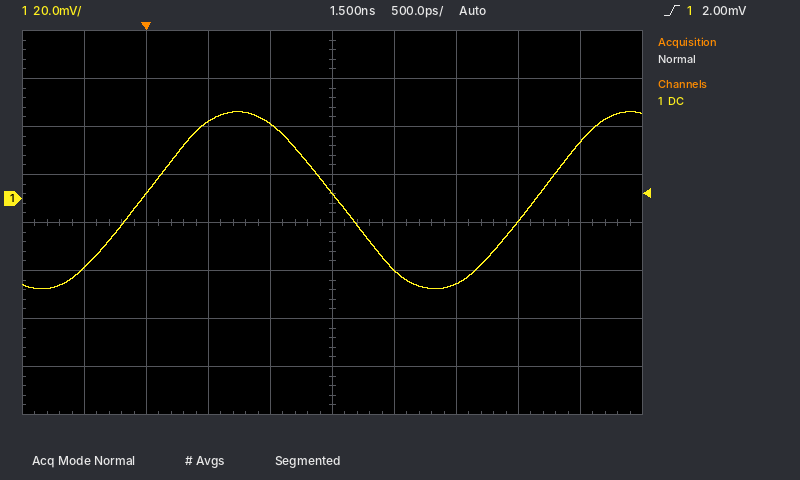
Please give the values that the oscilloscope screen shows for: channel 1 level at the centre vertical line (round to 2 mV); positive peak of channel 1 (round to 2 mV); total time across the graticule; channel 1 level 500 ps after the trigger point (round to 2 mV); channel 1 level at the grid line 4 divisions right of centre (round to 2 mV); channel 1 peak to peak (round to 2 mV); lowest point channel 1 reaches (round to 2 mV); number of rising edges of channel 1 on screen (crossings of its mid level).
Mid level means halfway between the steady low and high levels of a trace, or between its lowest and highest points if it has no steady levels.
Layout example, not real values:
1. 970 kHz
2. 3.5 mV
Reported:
1. 2 mV
2. 36 mV
3. 5 ns
4. 32 mV
5. 24 mV
6. 74 mV
7. -38 mV
8. 2
